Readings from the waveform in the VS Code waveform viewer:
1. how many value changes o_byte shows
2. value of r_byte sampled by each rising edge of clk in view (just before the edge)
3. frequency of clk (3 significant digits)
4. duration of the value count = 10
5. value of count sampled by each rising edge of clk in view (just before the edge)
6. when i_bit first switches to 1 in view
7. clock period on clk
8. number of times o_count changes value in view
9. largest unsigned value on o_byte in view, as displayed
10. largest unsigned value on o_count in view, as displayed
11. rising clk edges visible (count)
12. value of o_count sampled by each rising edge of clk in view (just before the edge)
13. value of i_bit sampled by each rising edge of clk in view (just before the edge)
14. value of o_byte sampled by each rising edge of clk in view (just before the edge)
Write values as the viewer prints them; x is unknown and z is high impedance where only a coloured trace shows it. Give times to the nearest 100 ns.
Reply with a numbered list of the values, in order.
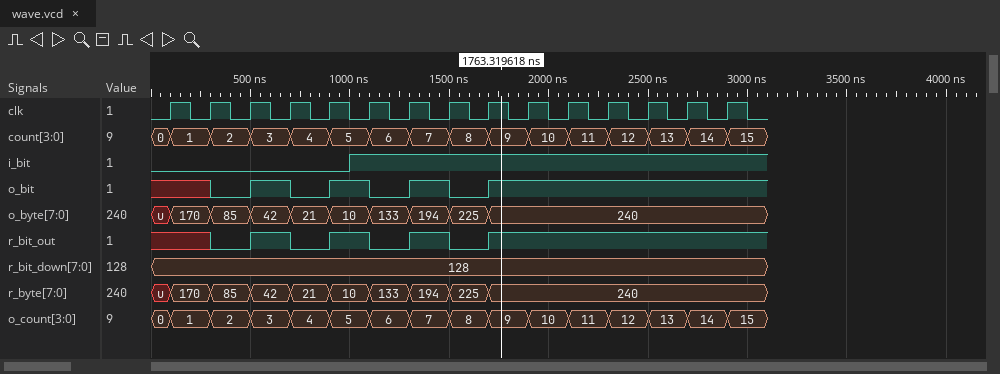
1. 9
2. u, 170, 85, 42, 21, 10, 133, 194, 225, 240, 240, 240, 240, 240, 240
3. 5.00 MHz
4. 200 ns
5. 0, 1, 2, 3, 4, 5, 6, 7, 8, 9, 10, 11, 12, 13, 14
6. 1000 ns
7. 200 ns
8. 15
9. 240
10. 15
11. 15
12. 0, 1, 2, 3, 4, 5, 6, 7, 8, 9, 10, 11, 12, 13, 14
13. 0 0 0 0 0 1 1 1 1 1 1 1 1 1 1
14. u, 170, 85, 42, 21, 10, 133, 194, 225, 240, 240, 240, 240, 240, 240
